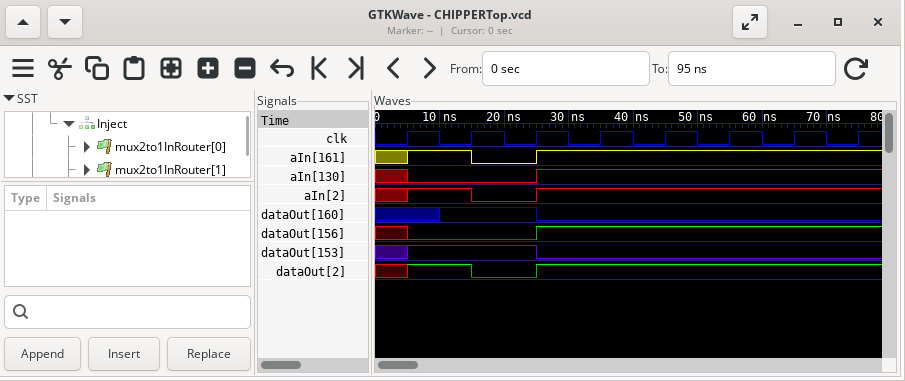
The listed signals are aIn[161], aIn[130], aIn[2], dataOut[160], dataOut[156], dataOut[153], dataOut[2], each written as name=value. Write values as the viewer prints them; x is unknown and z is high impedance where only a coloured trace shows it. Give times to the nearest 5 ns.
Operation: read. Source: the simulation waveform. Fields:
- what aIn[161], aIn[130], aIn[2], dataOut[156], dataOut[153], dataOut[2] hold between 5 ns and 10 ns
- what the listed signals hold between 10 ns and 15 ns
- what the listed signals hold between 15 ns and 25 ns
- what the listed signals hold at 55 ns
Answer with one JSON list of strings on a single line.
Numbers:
["aIn[161]=1, aIn[130]=0, aIn[2]=1, dataOut[156]=0, dataOut[153]=1, dataOut[2]=1", "aIn[161]=1, aIn[130]=0, aIn[2]=1, dataOut[160]=1, dataOut[156]=0, dataOut[153]=1, dataOut[2]=1", "aIn[161]=0, aIn[130]=0, aIn[2]=0, dataOut[160]=1, dataOut[156]=0, dataOut[153]=1, dataOut[2]=0", "aIn[161]=1, aIn[130]=1, aIn[2]=1, dataOut[160]=0, dataOut[156]=1, dataOut[153]=0, dataOut[2]=1"]
